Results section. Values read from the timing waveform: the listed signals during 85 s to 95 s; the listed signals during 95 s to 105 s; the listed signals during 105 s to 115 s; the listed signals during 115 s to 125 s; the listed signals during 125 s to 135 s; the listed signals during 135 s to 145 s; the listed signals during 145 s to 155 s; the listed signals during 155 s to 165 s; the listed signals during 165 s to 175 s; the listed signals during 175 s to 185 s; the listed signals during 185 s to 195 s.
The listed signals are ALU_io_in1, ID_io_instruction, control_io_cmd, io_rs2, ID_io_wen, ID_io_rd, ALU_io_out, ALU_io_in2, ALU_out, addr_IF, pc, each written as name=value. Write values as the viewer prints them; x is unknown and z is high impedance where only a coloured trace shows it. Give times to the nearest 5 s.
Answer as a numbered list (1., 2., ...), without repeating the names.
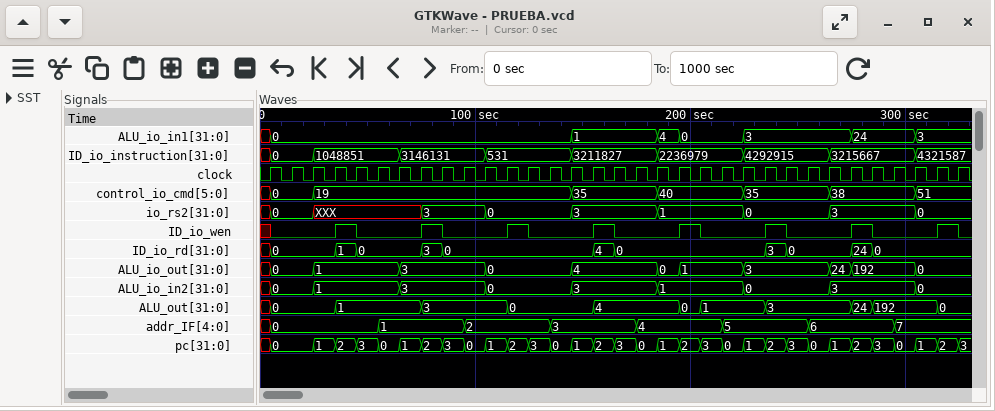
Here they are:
1. ALU_io_in1=0, ID_io_instruction=3146131, control_io_cmd=19, io_rs2=3, ID_io_wen=0, ID_io_rd=0, ALU_io_out=3, ALU_io_in2=3, ALU_out=3, addr_IF=1, pc=3
2. ALU_io_in1=0, ID_io_instruction=3146131, control_io_cmd=19, io_rs2=3, ID_io_wen=0, ID_io_rd=0, ALU_io_out=3, ALU_io_in2=3, ALU_out=3, addr_IF=2, pc=0
3. ALU_io_in1=0, ID_io_instruction=531, control_io_cmd=19, io_rs2=0, ID_io_wen=0, ID_io_rd=0, ALU_io_out=0, ALU_io_in2=0, ALU_out=3, addr_IF=2, pc=1
4. ALU_io_in1=0, ID_io_instruction=531, control_io_cmd=19, io_rs2=0, ID_io_wen=1, ID_io_rd=0, ALU_io_out=0, ALU_io_in2=0, ALU_out=0, addr_IF=2, pc=2
5. ALU_io_in1=0, ID_io_instruction=531, control_io_cmd=19, io_rs2=0, ID_io_wen=0, ID_io_rd=0, ALU_io_out=0, ALU_io_in2=0, ALU_out=0, addr_IF=2, pc=3
6. ALU_io_in1=0, ID_io_instruction=531, control_io_cmd=19, io_rs2=0, ID_io_wen=0, ID_io_rd=0, ALU_io_out=0, ALU_io_in2=0, ALU_out=0, addr_IF=3, pc=0
7. ALU_io_in1=1, ID_io_instruction=3211827, control_io_cmd=35, io_rs2=3, ID_io_wen=0, ID_io_rd=0, ALU_io_out=4, ALU_io_in2=3, ALU_out=0, addr_IF=3, pc=1
8. ALU_io_in1=1, ID_io_instruction=3211827, control_io_cmd=35, io_rs2=3, ID_io_wen=1, ID_io_rd=4, ALU_io_out=4, ALU_io_in2=3, ALU_out=4, addr_IF=3, pc=2
9. ALU_io_in1=1, ID_io_instruction=3211827, control_io_cmd=35, io_rs2=3, ID_io_wen=0, ID_io_rd=0, ALU_io_out=4, ALU_io_in2=3, ALU_out=4, addr_IF=3, pc=3
10. ALU_io_in1=1, ID_io_instruction=3211827, control_io_cmd=35, io_rs2=3, ID_io_wen=0, ID_io_rd=0, ALU_io_out=4, ALU_io_in2=3, ALU_out=4, addr_IF=4, pc=0
11. ALU_io_in1=4, ID_io_instruction=2236979, control_io_cmd=40, io_rs2=1, ID_io_wen=0, ID_io_rd=0, ALU_io_out=0, ALU_io_in2=1, ALU_out=4, addr_IF=4, pc=1
